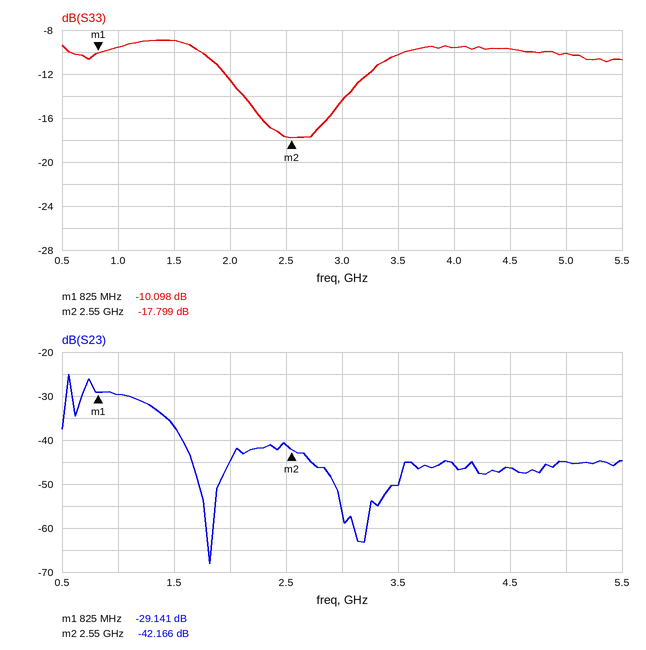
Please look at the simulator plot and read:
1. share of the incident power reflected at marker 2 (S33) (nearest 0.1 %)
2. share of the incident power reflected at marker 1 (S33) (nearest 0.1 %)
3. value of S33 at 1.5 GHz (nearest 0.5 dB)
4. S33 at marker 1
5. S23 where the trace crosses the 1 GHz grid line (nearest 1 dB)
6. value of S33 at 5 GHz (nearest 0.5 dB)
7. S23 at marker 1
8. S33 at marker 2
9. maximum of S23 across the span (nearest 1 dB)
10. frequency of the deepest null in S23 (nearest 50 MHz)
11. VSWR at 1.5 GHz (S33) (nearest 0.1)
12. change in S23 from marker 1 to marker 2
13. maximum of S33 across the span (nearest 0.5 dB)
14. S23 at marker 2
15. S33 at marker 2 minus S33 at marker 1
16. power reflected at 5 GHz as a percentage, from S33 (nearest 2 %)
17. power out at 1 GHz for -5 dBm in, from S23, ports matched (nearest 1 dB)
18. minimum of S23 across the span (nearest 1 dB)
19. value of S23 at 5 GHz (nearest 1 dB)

1.7 %
9.8 %
-9.0 dB
-10.098 dB
-30 dB
-10.0 dB
-29.141 dB
-17.799 dB
-25 dB
1.80 GHz
2.1
-13.025 dB
-9.0 dB
-42.166 dB
-7.701 dB
10 %
-35 dBm
-68 dB
-45 dB
